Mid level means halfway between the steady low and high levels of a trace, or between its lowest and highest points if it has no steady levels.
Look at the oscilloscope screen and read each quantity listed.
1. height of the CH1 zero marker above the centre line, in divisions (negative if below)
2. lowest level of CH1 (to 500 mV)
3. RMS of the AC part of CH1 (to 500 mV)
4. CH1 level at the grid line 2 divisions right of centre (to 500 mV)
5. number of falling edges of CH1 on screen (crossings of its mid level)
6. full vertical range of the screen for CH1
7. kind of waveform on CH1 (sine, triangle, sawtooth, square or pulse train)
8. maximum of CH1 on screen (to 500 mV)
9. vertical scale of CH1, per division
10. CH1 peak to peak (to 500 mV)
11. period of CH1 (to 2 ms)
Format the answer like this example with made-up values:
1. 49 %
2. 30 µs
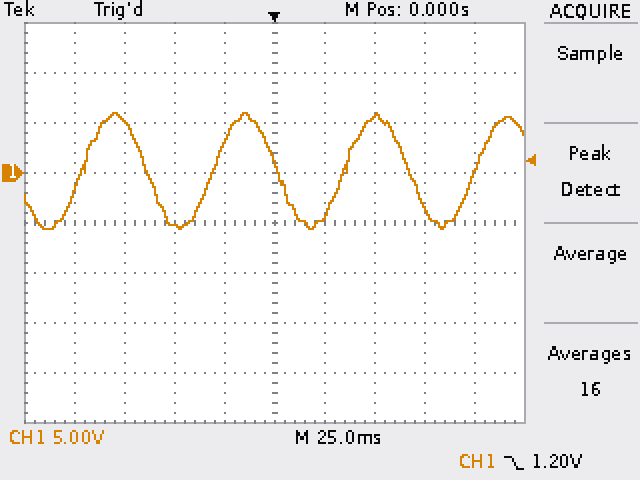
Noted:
1. +1.0 div
2. -5.5 V
3. 4.0 V
4. 5.5 V
5. 3
6. 40 V
7. sine
8. 6.0 V
9. 5 V
10. 11.5 V
11. 66 ms
